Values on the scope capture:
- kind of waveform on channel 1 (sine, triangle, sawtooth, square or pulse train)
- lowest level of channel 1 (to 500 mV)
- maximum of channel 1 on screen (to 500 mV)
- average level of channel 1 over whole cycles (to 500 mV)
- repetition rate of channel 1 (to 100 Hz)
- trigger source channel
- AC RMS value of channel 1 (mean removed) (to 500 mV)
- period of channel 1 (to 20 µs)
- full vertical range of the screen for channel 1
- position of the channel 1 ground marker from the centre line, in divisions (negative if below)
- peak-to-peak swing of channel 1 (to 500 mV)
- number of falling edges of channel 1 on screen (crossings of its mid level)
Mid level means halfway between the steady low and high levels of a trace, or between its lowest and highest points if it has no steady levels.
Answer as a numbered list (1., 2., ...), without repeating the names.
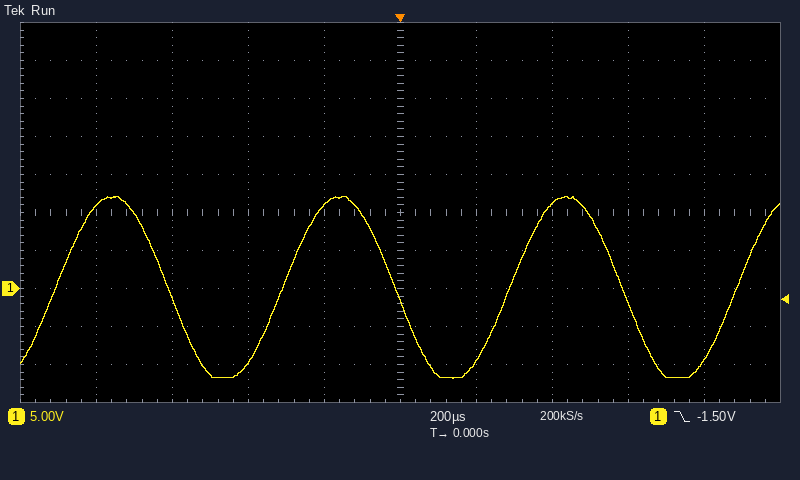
1. sine
2. -12.0 V
3. 12.0 V
4. 0.0 V
5. 1.7 kHz
6. channel 1
7. 8.5 V
8. 600 µs
9. 50 V
10. -2.0 div
11. 24.0 V
12. 3
